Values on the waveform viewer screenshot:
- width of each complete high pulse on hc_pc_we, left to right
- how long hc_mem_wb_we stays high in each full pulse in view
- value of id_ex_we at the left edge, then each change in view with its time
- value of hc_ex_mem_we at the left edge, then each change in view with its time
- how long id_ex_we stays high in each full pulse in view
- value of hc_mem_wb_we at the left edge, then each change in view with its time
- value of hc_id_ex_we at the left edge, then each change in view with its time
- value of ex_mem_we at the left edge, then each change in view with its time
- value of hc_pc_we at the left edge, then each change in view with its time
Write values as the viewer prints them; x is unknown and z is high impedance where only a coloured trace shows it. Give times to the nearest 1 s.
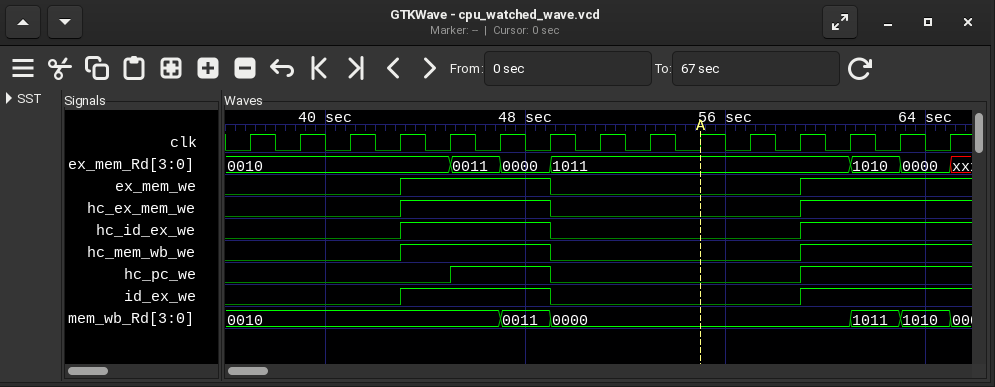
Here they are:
4 s
6 s
0, 1 at 43 s, 0 at 49 s, 1 at 59 s
0, 1 at 43 s, 0 at 49 s, 1 at 59 s
6 s
0, 1 at 43 s, 0 at 49 s, 1 at 59 s
0, 1 at 43 s, 0 at 49 s, 1 at 59 s
0, 1 at 43 s, 0 at 49 s, 1 at 59 s
0, 1 at 45 s, 0 at 49 s, 1 at 59 s
